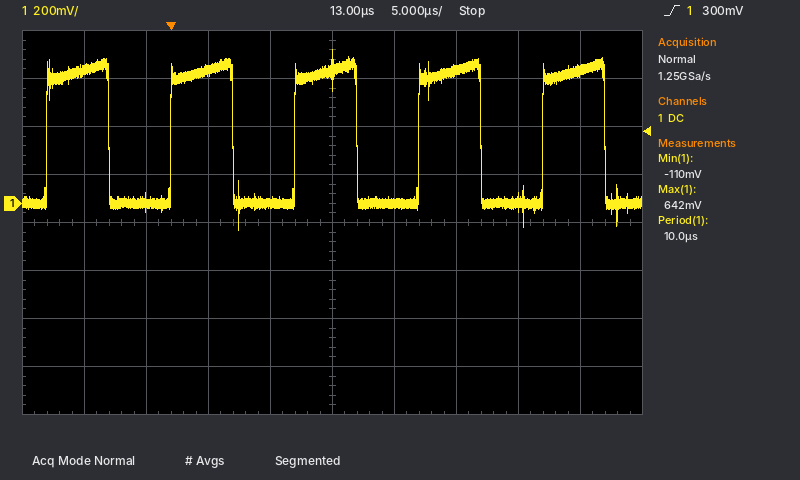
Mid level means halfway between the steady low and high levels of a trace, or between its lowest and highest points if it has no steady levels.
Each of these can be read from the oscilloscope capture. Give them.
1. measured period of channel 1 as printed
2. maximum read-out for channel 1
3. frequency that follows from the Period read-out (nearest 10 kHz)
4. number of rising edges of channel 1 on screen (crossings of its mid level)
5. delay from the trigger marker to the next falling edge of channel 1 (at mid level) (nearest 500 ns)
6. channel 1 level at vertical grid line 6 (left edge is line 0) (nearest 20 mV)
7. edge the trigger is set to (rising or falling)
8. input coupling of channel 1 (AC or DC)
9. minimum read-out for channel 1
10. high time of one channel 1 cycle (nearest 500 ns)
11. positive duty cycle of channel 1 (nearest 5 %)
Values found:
10.0 µs
642 mV
100 kHz
5
5.0 µs
0 mV
rising
DC
-110 mV
5.0 µs
50 %
